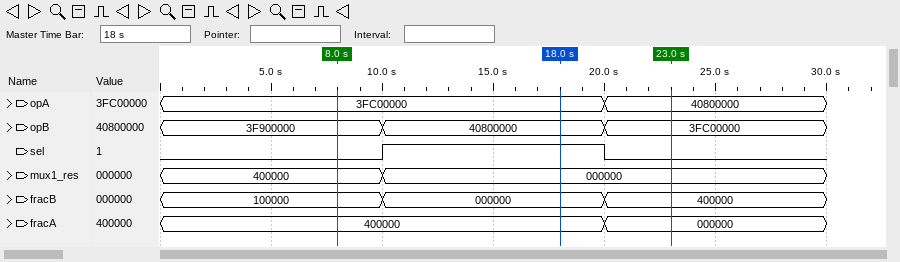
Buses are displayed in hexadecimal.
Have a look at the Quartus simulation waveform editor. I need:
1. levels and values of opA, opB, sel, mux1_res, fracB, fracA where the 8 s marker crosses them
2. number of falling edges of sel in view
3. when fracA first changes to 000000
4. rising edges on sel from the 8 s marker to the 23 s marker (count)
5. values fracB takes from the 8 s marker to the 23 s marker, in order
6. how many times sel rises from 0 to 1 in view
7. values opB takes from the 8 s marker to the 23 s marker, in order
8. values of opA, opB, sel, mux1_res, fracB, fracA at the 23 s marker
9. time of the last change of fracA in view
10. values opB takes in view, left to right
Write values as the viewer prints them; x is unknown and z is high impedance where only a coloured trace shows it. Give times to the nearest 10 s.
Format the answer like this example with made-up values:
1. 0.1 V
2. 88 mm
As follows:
1. opA=3FC00000, opB=3F900000, sel=0, mux1_res=400000, fracB=100000, fracA=400000
2. 1
3. 20 s
4. 1
5. 100000, 000000, 400000
6. 1
7. 3F900000, 40800000, 3FC00000
8. opA=40800000, opB=3FC00000, sel=0, mux1_res=000000, fracB=400000, fracA=000000
9. 20 s
10. 3F900000, 40800000, 3FC00000
